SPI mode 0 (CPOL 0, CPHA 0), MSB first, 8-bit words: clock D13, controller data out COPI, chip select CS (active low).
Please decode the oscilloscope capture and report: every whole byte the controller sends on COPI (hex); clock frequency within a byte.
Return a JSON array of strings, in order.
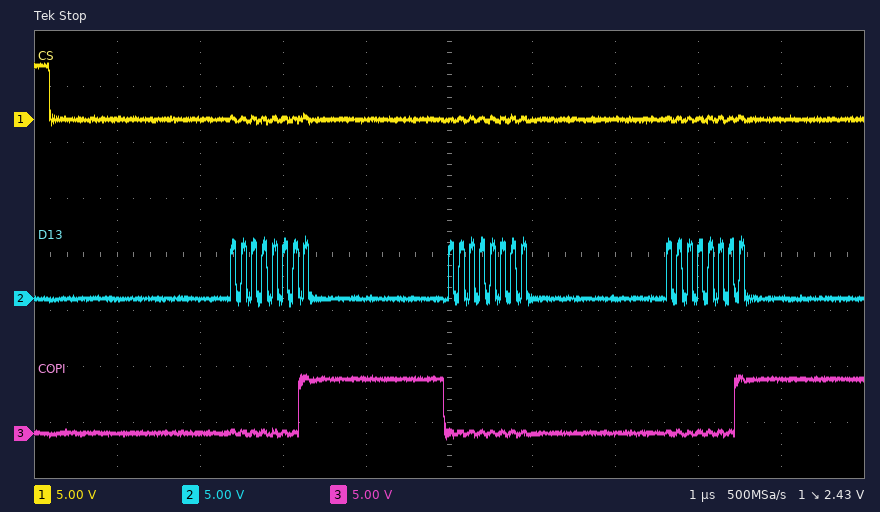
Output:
["0x01 0x00 0x01", "8 MHz"]
